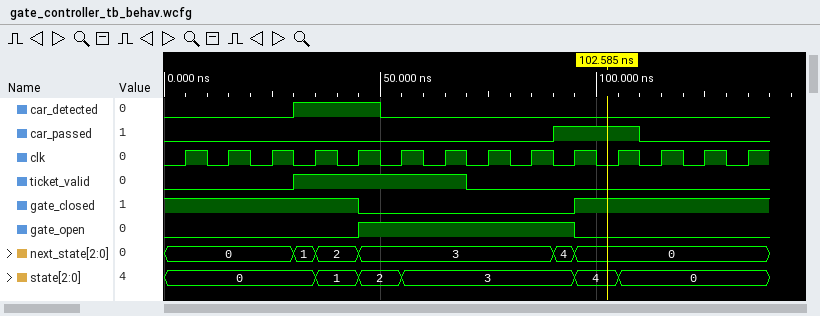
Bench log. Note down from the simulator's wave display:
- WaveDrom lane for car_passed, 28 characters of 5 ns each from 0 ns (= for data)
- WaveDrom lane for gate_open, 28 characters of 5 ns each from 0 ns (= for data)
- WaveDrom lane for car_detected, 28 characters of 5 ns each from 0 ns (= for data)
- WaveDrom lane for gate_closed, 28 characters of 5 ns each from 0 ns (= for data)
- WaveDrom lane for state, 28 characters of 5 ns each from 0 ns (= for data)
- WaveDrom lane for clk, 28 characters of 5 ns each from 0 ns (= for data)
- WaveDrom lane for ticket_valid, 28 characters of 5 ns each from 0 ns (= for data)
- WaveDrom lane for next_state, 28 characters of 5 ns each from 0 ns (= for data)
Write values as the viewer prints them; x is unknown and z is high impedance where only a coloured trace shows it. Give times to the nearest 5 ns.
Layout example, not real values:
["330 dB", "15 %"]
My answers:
["{name: 'car_passed', wave: '0.................1...0.....'}", "{name: 'gate_open', wave: '0........1.........0........'}", "{name: 'car_detected', wave: '0.....1...0.................'}", "{name: 'gate_closed', wave: '1........0.........1........'}", "{name: 'state', wave: '=......=.=.=.......=.=......', data: '0 1 2 3 4 0'}", "{name: 'clk', wave: '0101010101010101010101010101'}", "{name: 'ticket_valid', wave: '0.....1.......0.............'}", "{name: 'next_state', wave: '=.....==.=........==........', data: '0 1 2 3 4 0'}"]
